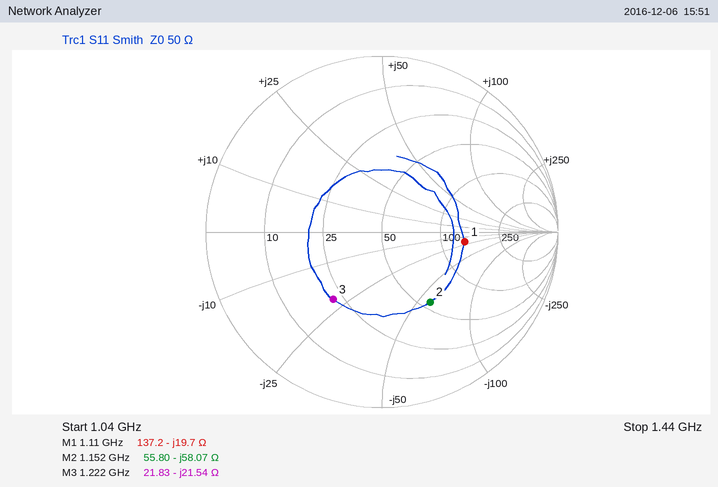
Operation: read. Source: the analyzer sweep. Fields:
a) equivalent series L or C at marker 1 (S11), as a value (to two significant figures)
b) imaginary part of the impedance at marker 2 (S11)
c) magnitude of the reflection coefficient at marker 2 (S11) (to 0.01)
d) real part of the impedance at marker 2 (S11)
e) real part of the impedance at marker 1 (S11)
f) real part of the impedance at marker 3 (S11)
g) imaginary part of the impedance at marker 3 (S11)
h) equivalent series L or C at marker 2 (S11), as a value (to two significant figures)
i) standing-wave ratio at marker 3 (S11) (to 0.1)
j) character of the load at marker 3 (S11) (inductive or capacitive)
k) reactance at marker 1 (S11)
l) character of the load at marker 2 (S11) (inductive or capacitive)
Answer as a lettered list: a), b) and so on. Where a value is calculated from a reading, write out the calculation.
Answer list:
a) C = 1/(2π × 1.11 GHz × 19.7 Ω) ≈ 7.3 pF
b) -58.07 Ω
c) 0.48
d) 55.80 Ω
e) 137.2 Ω
f) 21.83 Ω
g) -21.54 Ω
h) C = 1/(2π × 1.152 GHz × 58.07 Ω) ≈ 2.4 pF
i) 2.8
j) capacitive
k) -19.7 Ω
l) capacitive
